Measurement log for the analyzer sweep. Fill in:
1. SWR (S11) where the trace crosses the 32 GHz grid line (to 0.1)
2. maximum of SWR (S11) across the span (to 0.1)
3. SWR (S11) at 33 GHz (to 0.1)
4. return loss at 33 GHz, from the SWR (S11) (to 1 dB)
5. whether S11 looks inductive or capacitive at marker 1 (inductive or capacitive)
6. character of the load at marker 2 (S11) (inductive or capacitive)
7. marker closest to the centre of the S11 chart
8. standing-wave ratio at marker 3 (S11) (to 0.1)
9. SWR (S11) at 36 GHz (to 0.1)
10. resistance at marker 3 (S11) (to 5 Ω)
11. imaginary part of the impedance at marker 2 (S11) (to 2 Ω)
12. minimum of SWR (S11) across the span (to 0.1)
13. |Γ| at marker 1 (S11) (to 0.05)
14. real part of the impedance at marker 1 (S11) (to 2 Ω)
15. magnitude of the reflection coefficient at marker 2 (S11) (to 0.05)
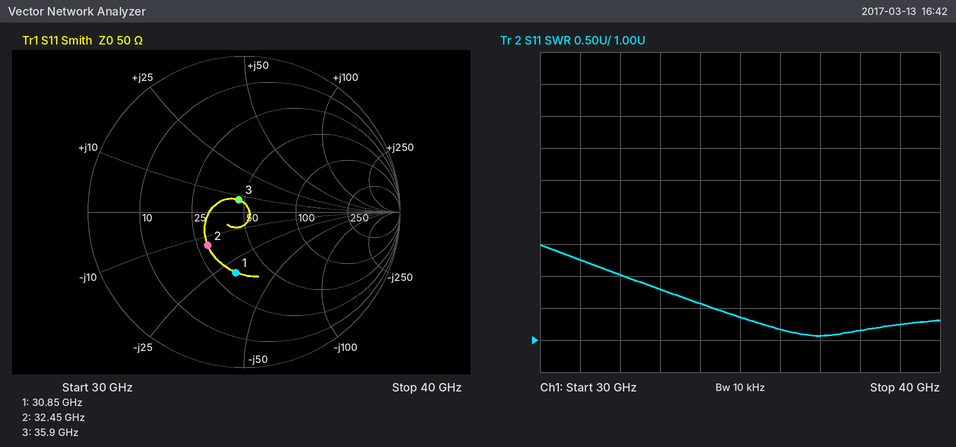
2.0
2.5
1.8
11 dB
capacitive
capacitive
marker 3
1.2
1.2
45 Ω
-14 Ω
1.1
0.40
34 Ω
0.30
